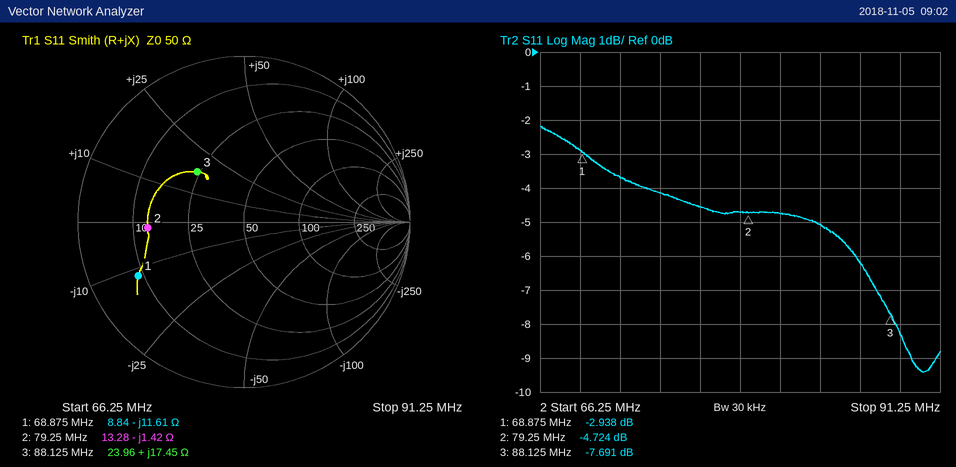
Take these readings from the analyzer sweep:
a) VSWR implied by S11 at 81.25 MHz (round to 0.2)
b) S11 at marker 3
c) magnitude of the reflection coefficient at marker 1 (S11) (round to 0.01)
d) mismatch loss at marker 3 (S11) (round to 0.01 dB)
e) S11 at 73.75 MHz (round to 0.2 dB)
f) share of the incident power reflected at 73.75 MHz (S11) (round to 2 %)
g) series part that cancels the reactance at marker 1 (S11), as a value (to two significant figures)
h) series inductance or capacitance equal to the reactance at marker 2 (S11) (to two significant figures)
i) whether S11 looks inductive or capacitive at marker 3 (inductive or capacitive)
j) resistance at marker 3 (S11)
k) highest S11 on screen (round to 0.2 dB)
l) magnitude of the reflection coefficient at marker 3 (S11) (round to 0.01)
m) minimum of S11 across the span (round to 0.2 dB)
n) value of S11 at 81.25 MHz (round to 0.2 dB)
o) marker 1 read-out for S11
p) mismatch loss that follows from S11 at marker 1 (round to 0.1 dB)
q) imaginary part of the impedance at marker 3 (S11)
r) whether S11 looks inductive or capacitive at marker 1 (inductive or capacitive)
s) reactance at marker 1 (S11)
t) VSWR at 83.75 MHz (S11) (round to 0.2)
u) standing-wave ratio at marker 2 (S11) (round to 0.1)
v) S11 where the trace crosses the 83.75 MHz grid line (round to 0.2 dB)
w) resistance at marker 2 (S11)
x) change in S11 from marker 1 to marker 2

3.8
-7.691 dB
0.71
0.81 dB
-4.2 dB
38 %
27 nH
1.4 nF
inductive
23.96 Ω
-2.2 dB
0.41
-9.4 dB
-4.8 dB
-2.938 dB
3.1 dB
+17.45 Ω
capacitive
-11.61 Ω
3.6
3.8
-5.0 dB
13.28 Ω
-1.786 dB
